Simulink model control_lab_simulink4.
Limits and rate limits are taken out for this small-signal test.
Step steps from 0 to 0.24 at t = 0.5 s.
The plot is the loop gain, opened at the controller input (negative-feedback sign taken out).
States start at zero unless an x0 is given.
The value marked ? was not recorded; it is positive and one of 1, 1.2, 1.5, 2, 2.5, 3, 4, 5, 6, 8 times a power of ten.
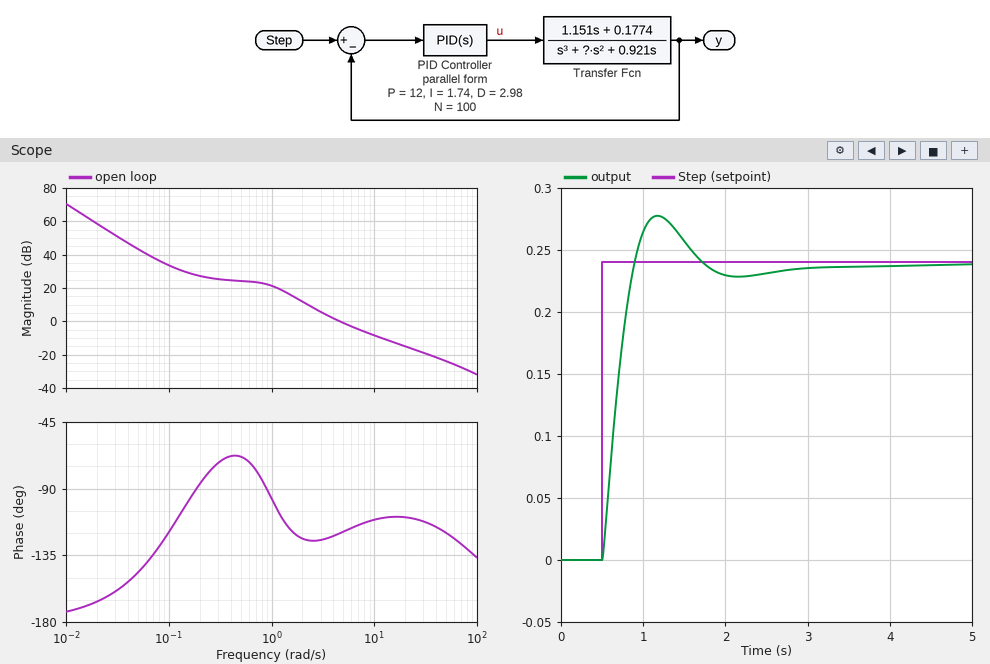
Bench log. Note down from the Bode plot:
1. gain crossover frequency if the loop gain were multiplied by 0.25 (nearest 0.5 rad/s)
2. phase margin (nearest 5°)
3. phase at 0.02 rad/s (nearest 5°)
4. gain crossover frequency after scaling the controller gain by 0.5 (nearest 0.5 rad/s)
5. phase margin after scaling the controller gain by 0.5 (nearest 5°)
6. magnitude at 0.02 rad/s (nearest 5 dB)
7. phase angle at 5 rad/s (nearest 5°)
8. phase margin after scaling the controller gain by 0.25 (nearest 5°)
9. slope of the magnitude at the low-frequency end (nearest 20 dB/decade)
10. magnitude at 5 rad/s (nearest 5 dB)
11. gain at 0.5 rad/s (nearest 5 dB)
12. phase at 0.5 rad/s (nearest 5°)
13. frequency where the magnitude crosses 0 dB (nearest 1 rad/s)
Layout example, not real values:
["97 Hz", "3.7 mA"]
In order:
["2.0 rad/s", "60°", "-165°", "3.0 rad/s", "55°", "60 dB", "-120°", "55°", "-40 dB/decade", "0 dB", "25 dB", "-70°", "5 rad/s"]
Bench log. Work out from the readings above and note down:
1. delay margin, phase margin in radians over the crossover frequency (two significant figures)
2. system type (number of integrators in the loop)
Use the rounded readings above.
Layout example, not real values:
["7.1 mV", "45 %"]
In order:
["0.21 s", "2"]
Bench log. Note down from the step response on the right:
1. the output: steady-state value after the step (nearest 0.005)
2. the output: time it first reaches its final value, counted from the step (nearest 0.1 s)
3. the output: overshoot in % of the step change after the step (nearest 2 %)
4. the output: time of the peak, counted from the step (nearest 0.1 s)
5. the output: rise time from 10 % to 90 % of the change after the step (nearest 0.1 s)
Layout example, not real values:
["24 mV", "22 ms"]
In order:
["0.240", "0.4 s", "16 %", "0.7 s", "0.3 s"]
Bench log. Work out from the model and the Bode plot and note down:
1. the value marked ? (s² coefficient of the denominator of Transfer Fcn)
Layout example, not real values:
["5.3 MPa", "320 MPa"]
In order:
["1.2"]
